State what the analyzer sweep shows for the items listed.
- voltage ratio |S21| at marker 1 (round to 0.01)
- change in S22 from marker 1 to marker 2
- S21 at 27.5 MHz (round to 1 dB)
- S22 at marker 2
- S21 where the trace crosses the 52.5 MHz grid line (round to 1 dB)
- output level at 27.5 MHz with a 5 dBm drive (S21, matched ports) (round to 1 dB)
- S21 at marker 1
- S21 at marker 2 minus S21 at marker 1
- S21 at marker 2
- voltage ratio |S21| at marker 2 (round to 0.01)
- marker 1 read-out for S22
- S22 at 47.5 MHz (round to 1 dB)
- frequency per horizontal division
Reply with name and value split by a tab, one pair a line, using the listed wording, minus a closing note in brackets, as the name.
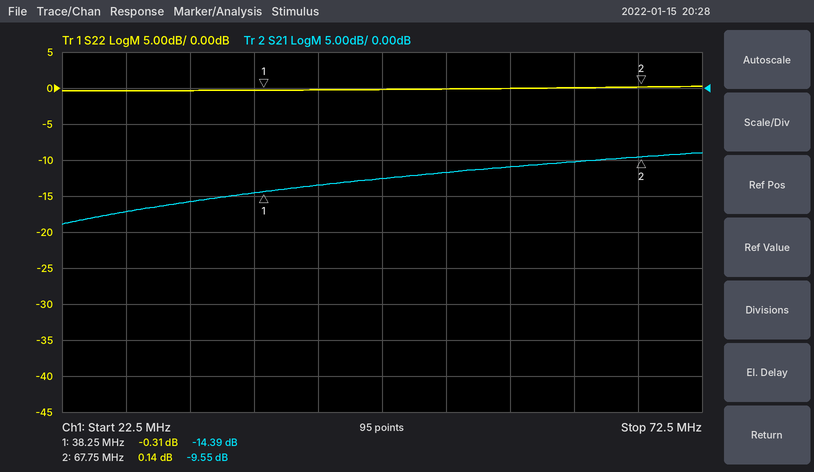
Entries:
voltage ratio |S21| at marker 1	0.19
change in S22 from marker 1 to marker 2	0.45 dB
S21 at 27.5 MHz	-17 dB
S22 at marker 2	0.14 dB
S21 where the trace crosses the 52.5 MHz grid line	-12 dB
output level at 27.5 MHz with a 5 dBm drive (S21, matched ports)	-12 dBm
S21 at marker 1	-14.39 dB
S21 at marker 2 minus S21 at marker 1	4.84 dB
S21 at marker 2	-9.55 dB
voltage ratio |S21| at marker 2	0.33
marker 1 read-out for S22	-0.31 dB
S22 at 47.5 MHz	0 dB
frequency per horizontal division	5 MHz
